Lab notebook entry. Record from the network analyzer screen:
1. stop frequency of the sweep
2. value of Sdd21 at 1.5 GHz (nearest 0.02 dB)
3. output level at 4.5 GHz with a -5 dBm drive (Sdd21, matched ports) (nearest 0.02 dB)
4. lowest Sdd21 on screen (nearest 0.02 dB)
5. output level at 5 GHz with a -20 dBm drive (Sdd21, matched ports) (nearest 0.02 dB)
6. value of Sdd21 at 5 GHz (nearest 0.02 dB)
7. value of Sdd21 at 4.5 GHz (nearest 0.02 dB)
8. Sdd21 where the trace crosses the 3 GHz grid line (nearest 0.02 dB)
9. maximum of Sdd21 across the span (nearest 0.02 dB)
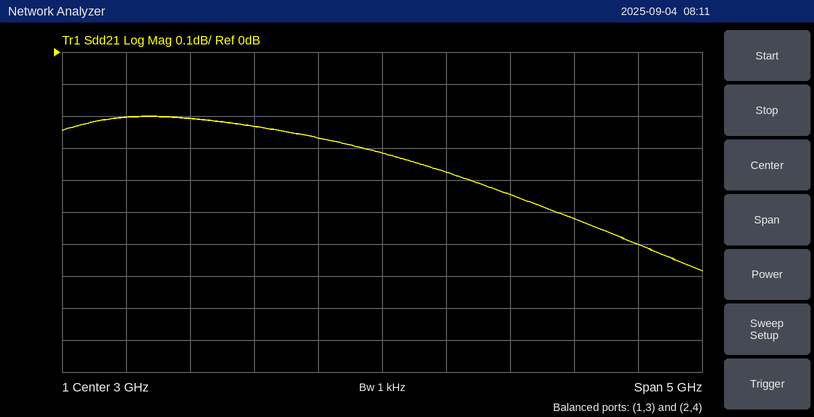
5.5 GHz
-0.20 dB
-5.52 dBm
-0.68 dB
-20.60 dBm
-0.60 dB
-0.52 dB
-0.32 dB
-0.20 dB
